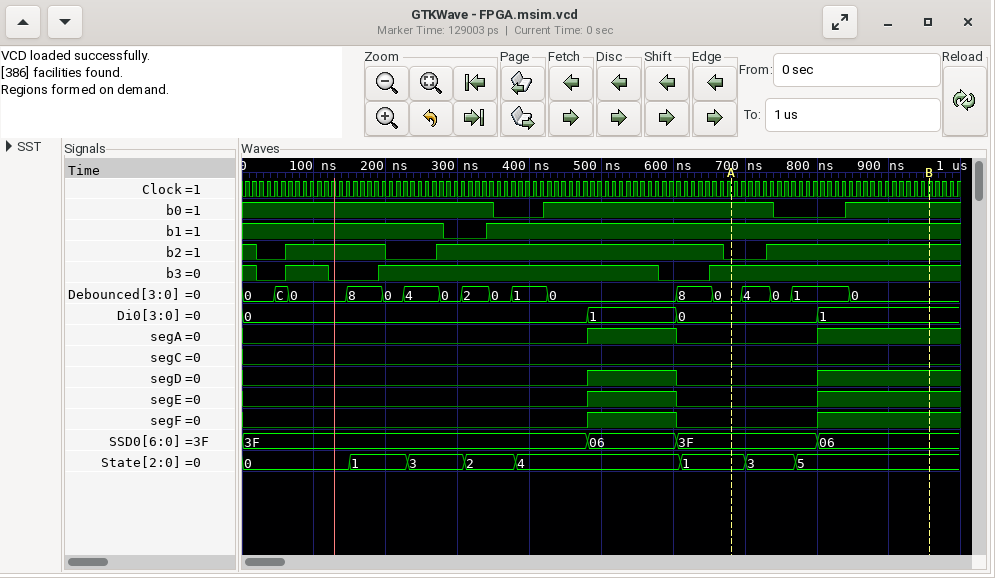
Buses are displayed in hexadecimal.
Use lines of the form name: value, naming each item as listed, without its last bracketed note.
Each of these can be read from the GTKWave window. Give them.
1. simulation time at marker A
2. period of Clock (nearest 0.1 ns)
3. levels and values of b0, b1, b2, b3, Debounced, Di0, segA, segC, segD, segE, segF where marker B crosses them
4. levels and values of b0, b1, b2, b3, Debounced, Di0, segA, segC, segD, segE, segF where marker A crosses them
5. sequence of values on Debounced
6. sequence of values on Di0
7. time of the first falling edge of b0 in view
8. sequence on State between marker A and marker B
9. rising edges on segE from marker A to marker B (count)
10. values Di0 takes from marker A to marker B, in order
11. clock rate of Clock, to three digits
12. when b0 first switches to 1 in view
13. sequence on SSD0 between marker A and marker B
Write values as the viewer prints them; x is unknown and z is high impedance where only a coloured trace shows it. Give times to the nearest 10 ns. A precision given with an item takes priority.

simulation time at marker A: 680 ns
period of Clock: 10 ns
levels and values of b0, b1, b2, b3, Debounced, Di0, segA, segC, segD, segE, segF where marker B crosses them: b0=1, b1=1, b2=1, b3=1, Debounced=0, Di0=1, segA=1, segC=0, segD=1, segE=1, segF=1
levels and values of b0, b1, b2, b3, Debounced, Di0, segA, segC, segD, segE, segF where marker A crosses them: b0=1, b1=1, b2=0, b3=1, Debounced=0, Di0=0, segA=0, segC=0, segD=0, segE=0, segF=0
sequence of values on Debounced: 0, C, 0, 8, 0, 4, 0, 2, 0, 1, 0, 8, 0, 4, 0, 1, 0
sequence of values on Di0: 0, 1, 0, 1
time of the first falling edge of b0 in view: 350 ns
sequence on State between marker A and marker B: 1, 3, 5
rising edges on segE from marker A to marker B: 1
values Di0 takes from marker A to marker B, in order: 0, 1
clock rate of Clock, to three digits: 100 MHz
when b0 first switches to 1 in view: 420 ns
sequence on SSD0 between marker A and marker B: 3F, 06
